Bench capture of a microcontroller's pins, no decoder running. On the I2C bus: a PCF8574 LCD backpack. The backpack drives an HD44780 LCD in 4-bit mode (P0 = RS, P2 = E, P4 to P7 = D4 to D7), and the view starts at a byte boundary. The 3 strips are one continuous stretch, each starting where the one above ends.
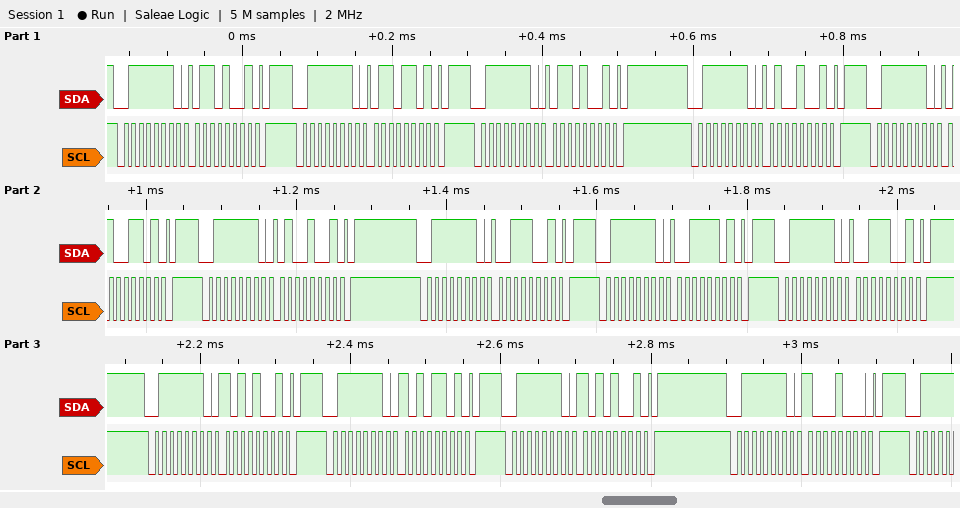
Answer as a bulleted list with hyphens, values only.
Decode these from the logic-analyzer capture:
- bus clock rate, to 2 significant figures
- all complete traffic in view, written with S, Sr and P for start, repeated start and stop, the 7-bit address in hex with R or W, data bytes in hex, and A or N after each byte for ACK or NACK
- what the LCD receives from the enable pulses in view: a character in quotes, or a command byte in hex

- 100 kHz
- S 3FW A 69 A P S 3FW A 6D A P S 3FW A 69 A P S 3FW A 49 A P S 3FW A 4D A P S 3FW A 49 A P S 3FW A 39 A P S 3FW A 3D A P S 3FW A 39 A P S 3FW A A9 A P S 3FW A AD A P S 3FW A A9 A P S 3FW A 88 A P
- 'd' ':'
